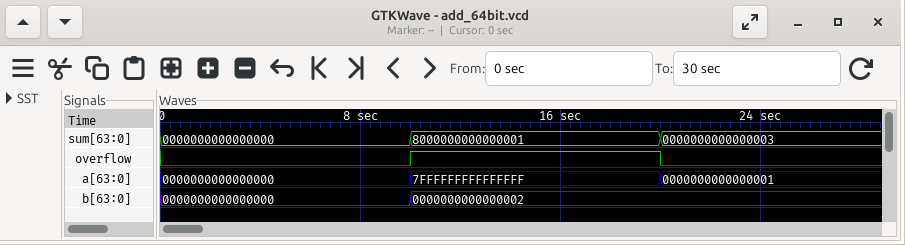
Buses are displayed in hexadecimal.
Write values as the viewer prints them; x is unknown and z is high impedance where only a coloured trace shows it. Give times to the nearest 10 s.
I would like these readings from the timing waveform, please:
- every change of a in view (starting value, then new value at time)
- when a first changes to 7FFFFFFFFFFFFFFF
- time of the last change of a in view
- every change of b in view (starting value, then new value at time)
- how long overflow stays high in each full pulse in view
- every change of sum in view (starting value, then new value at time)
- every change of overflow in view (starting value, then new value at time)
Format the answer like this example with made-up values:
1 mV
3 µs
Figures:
0000000000000000, 7FFFFFFFFFFFFFFF at 10 s, 0000000000000001 at 20 s
10 s
20 s
0000000000000000, 0000000000000002 at 10 s
10 s
0000000000000000, 8000000000000001 at 10 s, 0000000000000003 at 20 s
0, 1 at 10 s, 0 at 20 s
